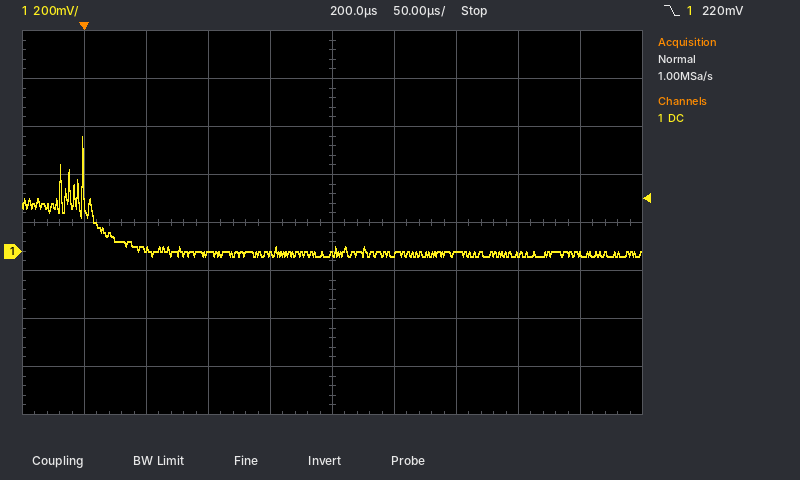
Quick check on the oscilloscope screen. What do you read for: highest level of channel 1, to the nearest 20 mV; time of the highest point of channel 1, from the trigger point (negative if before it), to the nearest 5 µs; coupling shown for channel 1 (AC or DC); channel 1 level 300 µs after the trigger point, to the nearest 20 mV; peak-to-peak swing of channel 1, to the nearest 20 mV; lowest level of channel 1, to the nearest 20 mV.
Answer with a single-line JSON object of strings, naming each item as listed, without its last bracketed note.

{"highest level of channel 1, to the nearest 20 mV": "480 mV", "time of the highest point of channel 1, from the trigger point (negative if before it), to the nearest 5 µs": "0 µs", "coupling shown for channel 1": "DC", "channel 1 level 300 µs after the trigger point, to the nearest 20 mV": "0 mV", "peak-to-peak swing of channel 1, to the nearest 20 mV": "500 mV", "lowest level of channel 1, to the nearest 20 mV": "-20 mV"}
